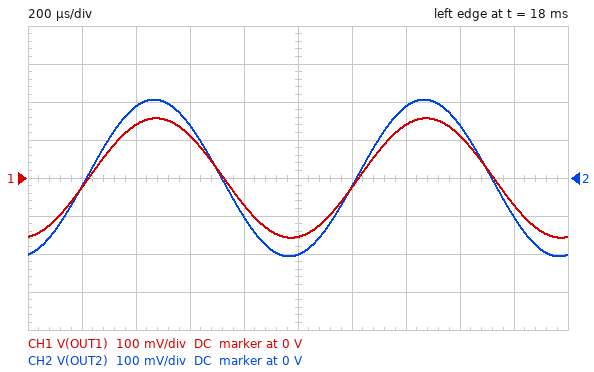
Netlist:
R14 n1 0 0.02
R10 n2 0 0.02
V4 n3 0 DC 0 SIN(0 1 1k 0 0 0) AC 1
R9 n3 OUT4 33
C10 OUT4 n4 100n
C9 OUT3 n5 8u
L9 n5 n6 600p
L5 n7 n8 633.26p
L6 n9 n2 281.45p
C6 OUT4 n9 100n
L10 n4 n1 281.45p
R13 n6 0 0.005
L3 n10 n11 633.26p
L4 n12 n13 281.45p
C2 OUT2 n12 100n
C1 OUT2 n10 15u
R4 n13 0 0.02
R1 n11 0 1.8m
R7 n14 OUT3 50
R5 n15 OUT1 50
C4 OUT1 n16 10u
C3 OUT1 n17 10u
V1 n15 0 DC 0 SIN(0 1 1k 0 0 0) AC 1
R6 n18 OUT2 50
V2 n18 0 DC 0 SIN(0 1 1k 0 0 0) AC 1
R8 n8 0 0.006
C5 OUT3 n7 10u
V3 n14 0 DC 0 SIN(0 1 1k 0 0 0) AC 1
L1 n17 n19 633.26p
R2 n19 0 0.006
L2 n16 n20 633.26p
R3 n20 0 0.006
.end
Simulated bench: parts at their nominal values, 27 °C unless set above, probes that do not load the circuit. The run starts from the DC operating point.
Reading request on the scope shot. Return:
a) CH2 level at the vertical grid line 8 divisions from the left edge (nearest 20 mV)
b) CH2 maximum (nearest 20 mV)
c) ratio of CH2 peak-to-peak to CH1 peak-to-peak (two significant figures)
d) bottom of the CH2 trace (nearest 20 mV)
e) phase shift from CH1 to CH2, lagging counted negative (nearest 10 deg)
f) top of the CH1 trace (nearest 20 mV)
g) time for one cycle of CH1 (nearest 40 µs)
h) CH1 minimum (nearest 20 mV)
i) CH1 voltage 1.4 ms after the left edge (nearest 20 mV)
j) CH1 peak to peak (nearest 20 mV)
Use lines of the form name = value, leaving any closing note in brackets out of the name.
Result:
CH2 level at the vertical grid line 8 divisions from the left edge = 140 mV
CH2 maximum = 200 mV
ratio of CH2 peak-to-peak to CH1 peak-to-peak = 1.3
bottom of the CH2 trace = -200 mV
phase shift from CH1 to CH2, lagging counted negative = 0 deg
top of the CH1 trace = 160 mV
time for one cycle of CH1 = 1.00 ms
CH1 minimum = -160 mV
CH1 voltage 1.4 ms after the left edge = 140 mV
CH1 peak to peak = 320 mV
